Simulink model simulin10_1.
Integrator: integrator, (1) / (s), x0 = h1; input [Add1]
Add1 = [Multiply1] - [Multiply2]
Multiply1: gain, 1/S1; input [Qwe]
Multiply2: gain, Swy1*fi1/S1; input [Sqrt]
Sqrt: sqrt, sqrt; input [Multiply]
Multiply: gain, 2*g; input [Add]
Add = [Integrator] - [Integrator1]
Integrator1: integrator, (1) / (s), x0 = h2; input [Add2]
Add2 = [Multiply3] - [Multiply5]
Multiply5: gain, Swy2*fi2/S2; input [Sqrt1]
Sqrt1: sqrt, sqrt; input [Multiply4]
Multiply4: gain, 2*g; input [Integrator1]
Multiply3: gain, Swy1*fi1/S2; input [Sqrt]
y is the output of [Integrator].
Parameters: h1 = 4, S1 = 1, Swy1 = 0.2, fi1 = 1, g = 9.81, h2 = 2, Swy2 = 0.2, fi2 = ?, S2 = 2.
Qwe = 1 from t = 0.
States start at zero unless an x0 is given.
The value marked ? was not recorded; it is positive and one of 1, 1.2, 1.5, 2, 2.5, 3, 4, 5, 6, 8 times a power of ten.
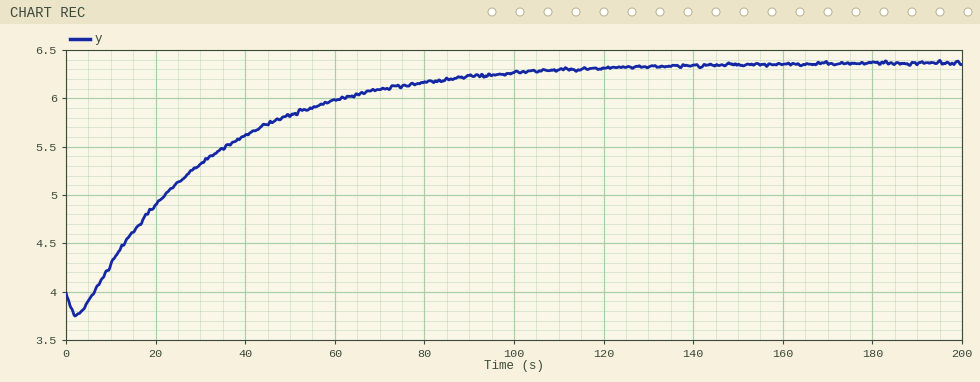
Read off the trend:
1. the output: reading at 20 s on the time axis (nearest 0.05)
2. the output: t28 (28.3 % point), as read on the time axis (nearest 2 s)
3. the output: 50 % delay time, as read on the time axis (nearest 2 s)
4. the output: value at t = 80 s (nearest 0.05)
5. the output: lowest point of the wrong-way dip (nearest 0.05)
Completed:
4.90
16 s
26 s
6.15
3.75
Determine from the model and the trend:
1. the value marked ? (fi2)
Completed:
0.5
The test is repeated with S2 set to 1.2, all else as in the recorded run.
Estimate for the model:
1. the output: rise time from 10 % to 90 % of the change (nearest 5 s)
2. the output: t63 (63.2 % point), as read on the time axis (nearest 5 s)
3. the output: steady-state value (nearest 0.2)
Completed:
50 s
25 s
6.4
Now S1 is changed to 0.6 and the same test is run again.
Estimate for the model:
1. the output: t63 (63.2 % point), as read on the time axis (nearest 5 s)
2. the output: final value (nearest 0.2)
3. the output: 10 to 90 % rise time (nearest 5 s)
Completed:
30 s
6.4
55 s
